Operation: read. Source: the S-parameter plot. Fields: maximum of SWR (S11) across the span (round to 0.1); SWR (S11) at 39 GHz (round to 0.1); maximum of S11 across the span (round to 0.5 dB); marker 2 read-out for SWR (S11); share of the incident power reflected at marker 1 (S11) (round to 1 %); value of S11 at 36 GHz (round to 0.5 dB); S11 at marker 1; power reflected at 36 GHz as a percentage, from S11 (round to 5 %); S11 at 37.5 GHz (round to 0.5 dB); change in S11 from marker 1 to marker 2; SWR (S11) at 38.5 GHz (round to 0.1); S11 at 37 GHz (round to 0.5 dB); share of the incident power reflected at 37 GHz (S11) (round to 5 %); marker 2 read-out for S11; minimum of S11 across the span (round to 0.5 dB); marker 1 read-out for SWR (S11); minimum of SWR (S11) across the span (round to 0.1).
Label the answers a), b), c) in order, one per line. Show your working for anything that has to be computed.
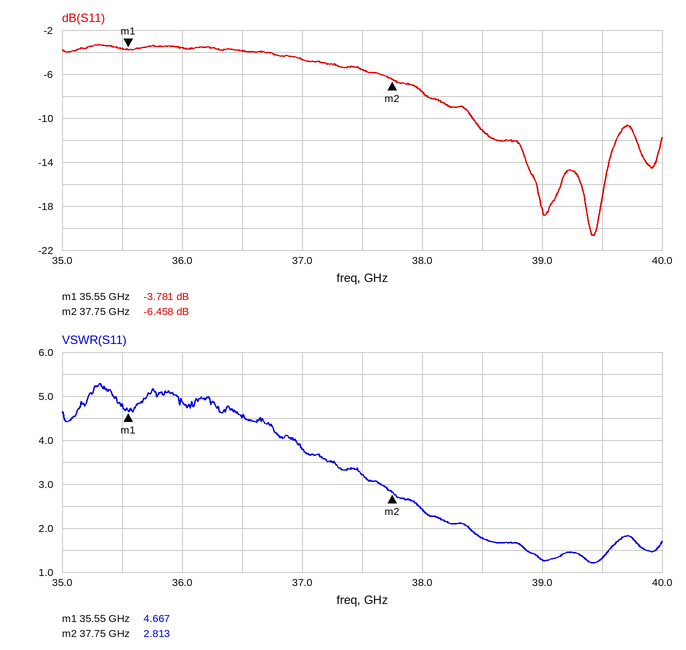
a) 5.3
b) 1.3
c) -3.5 dB
d) 2.813
e) 10^(-3.781/10) ≈ 42 %
f) -3.5 dB
g) -3.781 dB
h) 10^(-3.5/10) ≈ 45 %
i) -5.5 dB
j) -6.458 − (-3.781) = -2.677 dB
k) 1.8
l) -4.5 dB
m) 10^(-4.5/10) ≈ 35 %
n) -6.458 dB
o) -20.5 dB
p) 4.667
q) 1.2
